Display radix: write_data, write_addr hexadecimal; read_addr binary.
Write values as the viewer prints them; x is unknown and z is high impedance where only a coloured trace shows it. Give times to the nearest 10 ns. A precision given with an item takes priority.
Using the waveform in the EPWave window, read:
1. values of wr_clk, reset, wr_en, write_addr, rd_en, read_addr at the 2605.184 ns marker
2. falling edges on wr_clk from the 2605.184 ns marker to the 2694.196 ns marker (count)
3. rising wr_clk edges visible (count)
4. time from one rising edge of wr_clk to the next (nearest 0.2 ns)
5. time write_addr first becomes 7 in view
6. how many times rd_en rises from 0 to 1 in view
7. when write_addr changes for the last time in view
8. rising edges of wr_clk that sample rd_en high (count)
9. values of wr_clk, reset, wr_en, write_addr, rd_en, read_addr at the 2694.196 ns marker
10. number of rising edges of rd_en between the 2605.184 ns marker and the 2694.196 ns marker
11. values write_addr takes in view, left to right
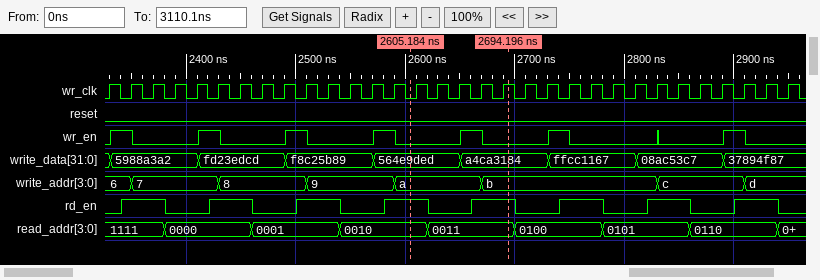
wr_clk=0, reset=0, wr_en=0, write_addr=a, rd_en=1, read_addr=0010
4
32
20 ns
2350 ns
8
2910 ns
16
wr_clk=1, reset=0, wr_en=0, write_addr=b, rd_en=1, read_addr=0011
1
6, 7, 8, 9, a, b, c, d
